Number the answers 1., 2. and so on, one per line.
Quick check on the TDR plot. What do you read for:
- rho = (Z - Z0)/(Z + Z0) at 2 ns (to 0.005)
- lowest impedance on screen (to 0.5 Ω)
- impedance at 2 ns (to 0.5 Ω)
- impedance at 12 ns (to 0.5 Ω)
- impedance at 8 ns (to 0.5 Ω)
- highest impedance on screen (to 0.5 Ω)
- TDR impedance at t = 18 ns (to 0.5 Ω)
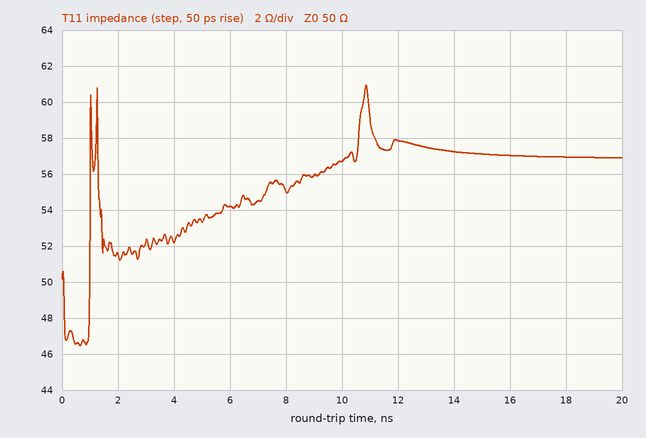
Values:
1. +0.015
2. 46.5 Ω
3. 51.5 Ω
4. 58.0 Ω
5. 55.0 Ω
6. 61.0 Ω
7. 57.0 Ω
